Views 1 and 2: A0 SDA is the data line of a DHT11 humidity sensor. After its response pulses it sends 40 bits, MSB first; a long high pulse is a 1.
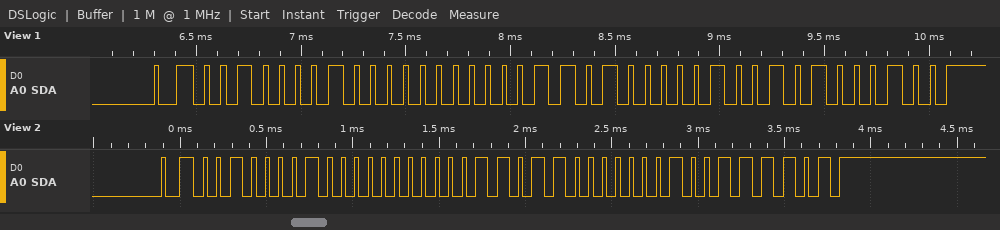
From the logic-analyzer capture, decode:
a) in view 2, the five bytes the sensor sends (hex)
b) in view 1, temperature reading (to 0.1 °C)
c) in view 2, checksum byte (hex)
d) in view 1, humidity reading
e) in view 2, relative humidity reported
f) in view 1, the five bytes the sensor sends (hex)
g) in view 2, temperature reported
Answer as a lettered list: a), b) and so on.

a) 21 00 1B 01 3D
b) 26.9 °C
c) 0x3D
d) 33 %
e) 33 %
f) 21 00 1A 09 44
g) 27.1 °C
